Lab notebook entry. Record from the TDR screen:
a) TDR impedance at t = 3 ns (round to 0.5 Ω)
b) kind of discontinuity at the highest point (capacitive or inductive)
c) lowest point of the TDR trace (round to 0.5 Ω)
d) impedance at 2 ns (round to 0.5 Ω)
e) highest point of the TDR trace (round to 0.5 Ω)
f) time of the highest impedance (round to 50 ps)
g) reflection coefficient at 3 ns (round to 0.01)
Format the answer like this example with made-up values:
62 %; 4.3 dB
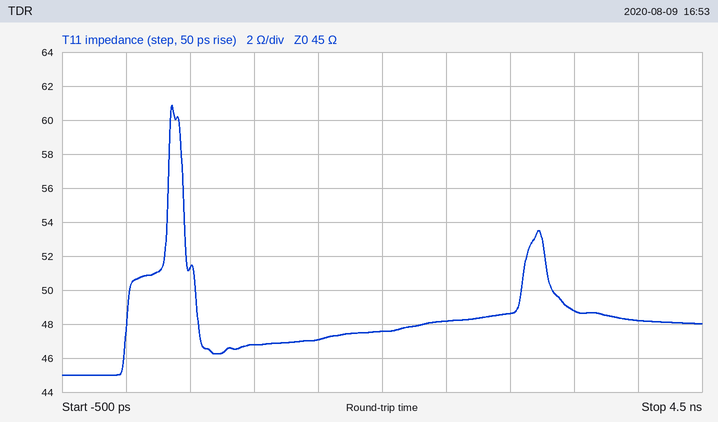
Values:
48.5 Ω; inductive; 45.0 Ω; 47.5 Ω; 61.0 Ω; 350 ps; +0.04
